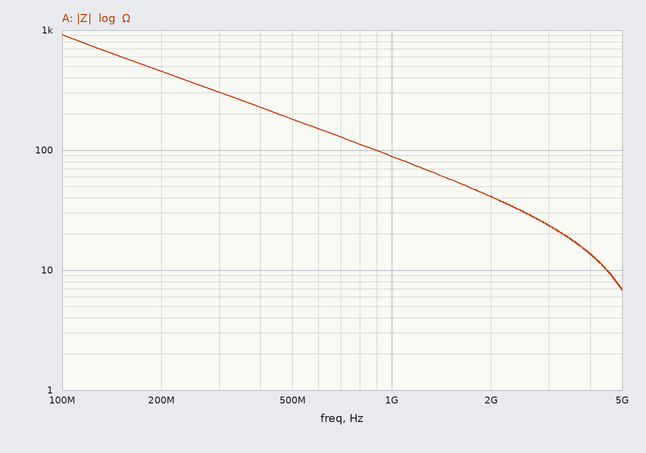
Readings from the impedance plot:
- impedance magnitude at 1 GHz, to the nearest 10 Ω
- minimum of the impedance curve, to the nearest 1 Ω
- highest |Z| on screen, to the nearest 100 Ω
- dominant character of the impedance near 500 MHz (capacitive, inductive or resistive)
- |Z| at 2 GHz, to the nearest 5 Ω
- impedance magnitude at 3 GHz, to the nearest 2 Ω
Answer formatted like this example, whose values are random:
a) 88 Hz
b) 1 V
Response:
a) 90 Ω
b) 7 Ω
c) 900 Ω
d) capacitive
e) 40 Ω
f) 24 Ω
